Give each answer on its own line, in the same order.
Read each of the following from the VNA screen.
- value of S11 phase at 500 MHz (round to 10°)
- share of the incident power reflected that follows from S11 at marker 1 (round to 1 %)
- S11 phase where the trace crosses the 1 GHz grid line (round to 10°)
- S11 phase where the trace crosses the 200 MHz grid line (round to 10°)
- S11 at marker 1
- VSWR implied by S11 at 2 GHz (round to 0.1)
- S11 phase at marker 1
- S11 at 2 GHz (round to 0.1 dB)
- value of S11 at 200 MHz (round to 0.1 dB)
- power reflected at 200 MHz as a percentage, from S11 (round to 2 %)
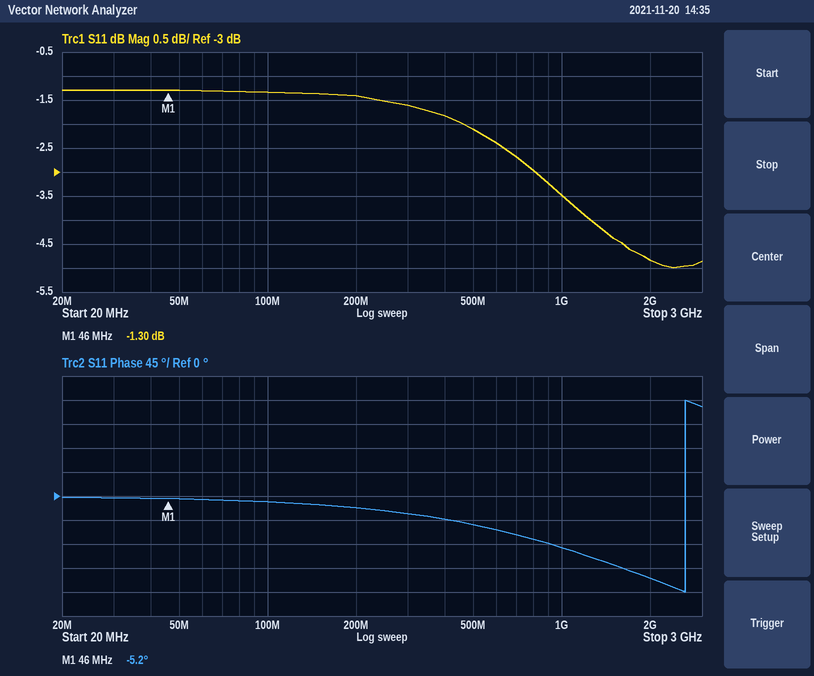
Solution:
-50°
74 %
-100°
-20°
-1.30 dB
3.7
-5.2°
-4.8 dB
-1.4 dB
72 %
